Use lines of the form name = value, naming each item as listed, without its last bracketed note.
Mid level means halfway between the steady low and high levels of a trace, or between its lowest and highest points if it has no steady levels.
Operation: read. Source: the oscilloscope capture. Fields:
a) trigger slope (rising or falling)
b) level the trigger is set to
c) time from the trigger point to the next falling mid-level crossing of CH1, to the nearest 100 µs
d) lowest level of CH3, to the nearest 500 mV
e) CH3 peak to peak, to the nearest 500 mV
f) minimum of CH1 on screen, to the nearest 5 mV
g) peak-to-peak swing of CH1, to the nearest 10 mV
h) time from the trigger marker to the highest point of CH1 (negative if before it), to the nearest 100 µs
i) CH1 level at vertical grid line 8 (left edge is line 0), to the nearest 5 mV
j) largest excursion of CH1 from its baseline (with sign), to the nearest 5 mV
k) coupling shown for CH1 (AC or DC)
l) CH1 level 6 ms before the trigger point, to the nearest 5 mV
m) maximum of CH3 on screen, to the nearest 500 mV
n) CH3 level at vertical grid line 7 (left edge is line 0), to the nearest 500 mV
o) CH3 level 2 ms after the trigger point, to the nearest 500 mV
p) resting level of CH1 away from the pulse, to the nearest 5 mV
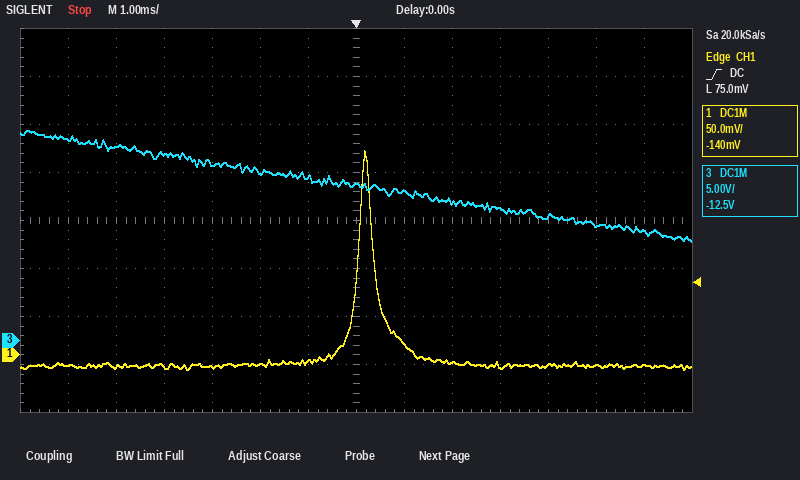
trigger slope = rising
level the trigger is set to = 75.0 mV
time from the trigger point to the next falling mid-level crossing of CH1, to the nearest 100 µs = 400 µs
lowest level of CH3, to the nearest 500 mV = 10.5 V
CH3 peak to peak, to the nearest 500 mV = 11.5 V
minimum of CH1 on screen, to the nearest 5 mV = -15 mV
peak-to-peak swing of CH1, to the nearest 10 mV = 230 mV
time from the trigger marker to the highest point of CH1 (negative if before it), to the nearest 100 µs = +200 µs
CH1 level at vertical grid line 8 (left edge is line 0), to the nearest 5 mV = 10 mV
largest excursion of CH1 from its baseline (with sign), to the nearest 5 mV = +225 mV
coupling shown for CH1 = DC
CH1 level 6 ms before the trigger point, to the nearest 5 mV = -10 mV
maximum of CH3 on screen, to the nearest 500 mV = 22.0 V
CH3 level at vertical grid line 7 (left edge is line 0), to the nearest 500 mV = 16.5 V
CH3 level 2 ms after the trigger point, to the nearest 500 mV = 14.5 V
resting level of CH1 away from the pulse, to the nearest 5 mV = -10 mV
